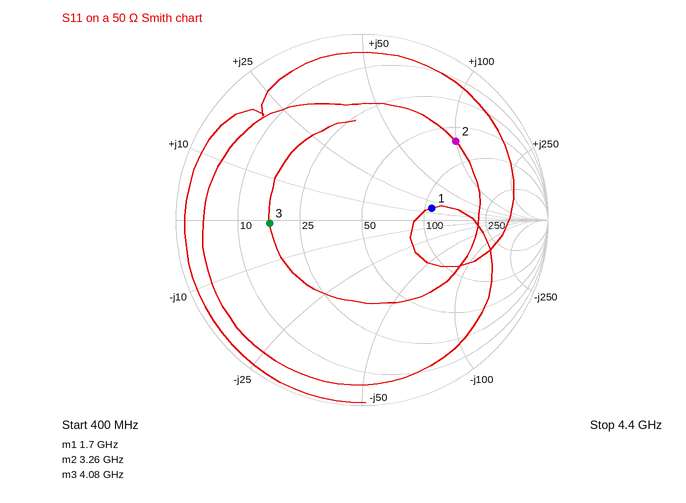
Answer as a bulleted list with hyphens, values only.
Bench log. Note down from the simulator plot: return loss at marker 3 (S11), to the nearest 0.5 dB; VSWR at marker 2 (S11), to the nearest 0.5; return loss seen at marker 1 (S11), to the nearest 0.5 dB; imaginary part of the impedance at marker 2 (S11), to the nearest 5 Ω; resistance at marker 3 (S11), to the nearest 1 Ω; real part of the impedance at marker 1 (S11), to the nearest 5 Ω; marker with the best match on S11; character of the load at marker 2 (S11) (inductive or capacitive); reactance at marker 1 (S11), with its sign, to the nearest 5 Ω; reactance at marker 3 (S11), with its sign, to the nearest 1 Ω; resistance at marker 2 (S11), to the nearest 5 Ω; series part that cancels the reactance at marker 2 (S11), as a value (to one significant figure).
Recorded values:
- 6.0 dB
- 5.0
- 8.5 dB
- +100 Ω
- 17 Ω
- 110 Ω
- marker 1
- inductive
- +15 Ω
- -1 Ω
- 65 Ω
- 500 fF
